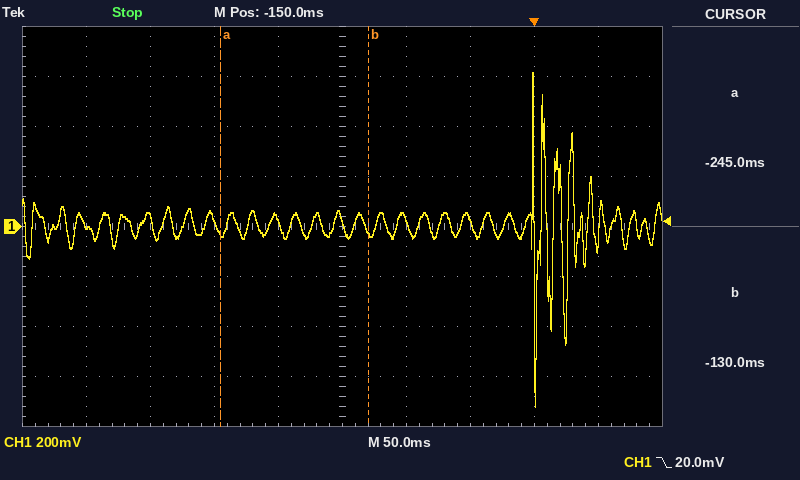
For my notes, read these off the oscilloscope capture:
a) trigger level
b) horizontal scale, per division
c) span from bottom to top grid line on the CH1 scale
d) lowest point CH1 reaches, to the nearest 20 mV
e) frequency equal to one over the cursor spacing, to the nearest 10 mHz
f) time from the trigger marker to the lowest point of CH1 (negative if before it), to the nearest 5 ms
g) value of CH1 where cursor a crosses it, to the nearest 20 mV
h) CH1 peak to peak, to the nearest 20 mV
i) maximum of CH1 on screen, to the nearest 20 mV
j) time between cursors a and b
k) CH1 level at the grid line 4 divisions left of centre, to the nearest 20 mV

20.0 mV
50 ms
1.6 V
-720 mV
8.70 Hz
0 ms
-20 mV
1.34 V
620 mV
115 ms
0 mV
